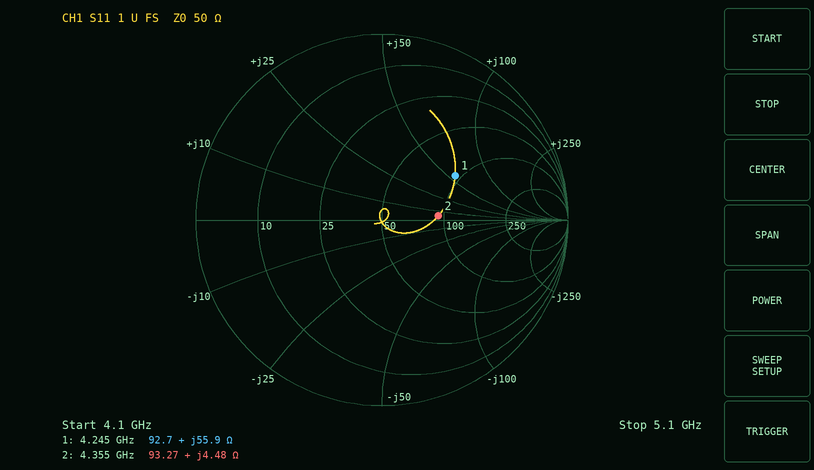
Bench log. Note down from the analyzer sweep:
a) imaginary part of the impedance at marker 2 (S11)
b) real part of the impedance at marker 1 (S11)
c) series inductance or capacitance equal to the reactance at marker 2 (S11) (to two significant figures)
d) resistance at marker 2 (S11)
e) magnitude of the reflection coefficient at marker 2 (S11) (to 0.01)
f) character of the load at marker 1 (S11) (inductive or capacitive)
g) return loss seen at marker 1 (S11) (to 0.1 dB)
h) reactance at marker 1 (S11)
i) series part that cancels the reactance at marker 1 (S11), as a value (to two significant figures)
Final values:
+4.48 Ω
92.7 Ω
160 pH
93.27 Ω
0.30
inductive
6.8 dB
+55.9 Ω
670 fF
